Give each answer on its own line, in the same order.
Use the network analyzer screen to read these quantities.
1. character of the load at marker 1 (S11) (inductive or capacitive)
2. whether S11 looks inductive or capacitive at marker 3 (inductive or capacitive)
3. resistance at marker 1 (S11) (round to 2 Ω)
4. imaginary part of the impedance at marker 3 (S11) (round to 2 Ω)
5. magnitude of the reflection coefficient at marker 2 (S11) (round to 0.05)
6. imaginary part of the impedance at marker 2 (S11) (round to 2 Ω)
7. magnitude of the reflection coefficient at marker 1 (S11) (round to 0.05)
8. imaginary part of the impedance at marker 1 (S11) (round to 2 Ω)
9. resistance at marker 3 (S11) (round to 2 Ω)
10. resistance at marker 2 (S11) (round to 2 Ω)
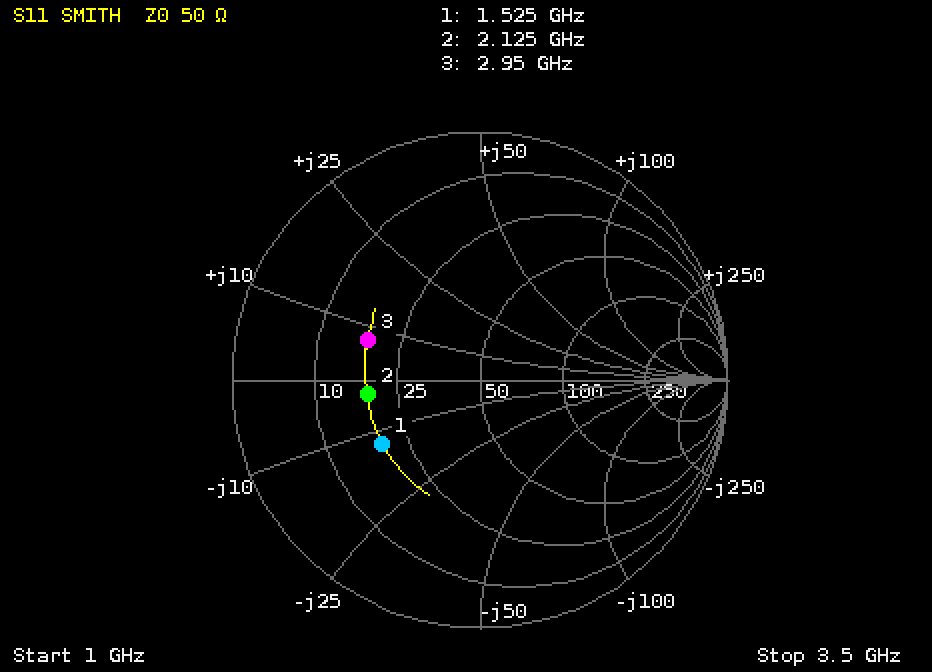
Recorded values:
capacitive
inductive
20 Ω
+8 Ω
0.45
-2 Ω
0.45
-12 Ω
18 Ω
18 Ω
